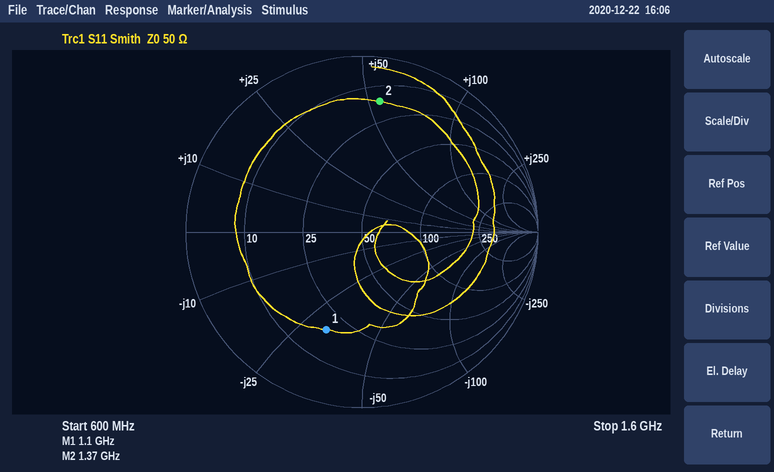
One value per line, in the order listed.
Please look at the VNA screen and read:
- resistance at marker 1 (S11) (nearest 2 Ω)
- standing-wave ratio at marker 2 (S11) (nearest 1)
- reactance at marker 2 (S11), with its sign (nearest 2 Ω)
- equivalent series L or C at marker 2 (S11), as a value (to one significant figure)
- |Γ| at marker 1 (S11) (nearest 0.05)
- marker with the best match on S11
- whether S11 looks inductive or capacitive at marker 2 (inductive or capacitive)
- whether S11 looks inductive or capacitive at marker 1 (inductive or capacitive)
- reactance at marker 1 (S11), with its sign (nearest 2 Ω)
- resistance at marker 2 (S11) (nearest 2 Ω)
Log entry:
18 Ω
7
+54 Ω
6 nH
0.60
marker 1
inductive
capacitive
-32 Ω
16 Ω
